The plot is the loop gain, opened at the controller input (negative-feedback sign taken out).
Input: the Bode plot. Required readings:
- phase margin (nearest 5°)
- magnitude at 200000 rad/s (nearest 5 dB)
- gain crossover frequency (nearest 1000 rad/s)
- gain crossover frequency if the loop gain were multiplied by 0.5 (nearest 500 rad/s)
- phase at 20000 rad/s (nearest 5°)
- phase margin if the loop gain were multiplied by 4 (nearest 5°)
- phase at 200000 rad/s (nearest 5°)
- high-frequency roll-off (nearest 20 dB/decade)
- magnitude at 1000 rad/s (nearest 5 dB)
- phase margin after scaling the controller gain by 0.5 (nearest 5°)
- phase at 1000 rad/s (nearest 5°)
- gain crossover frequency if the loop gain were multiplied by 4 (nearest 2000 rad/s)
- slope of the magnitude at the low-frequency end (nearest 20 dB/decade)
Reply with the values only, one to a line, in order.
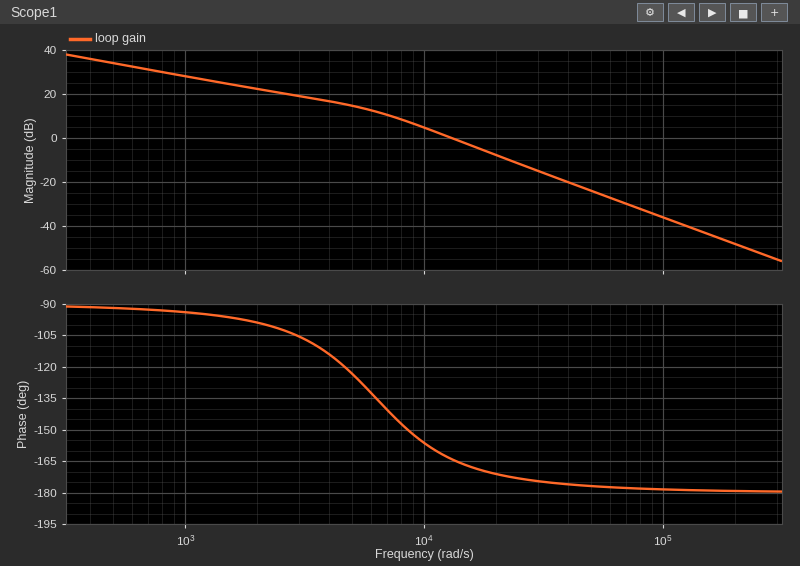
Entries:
15°
-50 dB
13000 rad/s
9500 rad/s
-170°
5°
-180°
-40 dB/decade
30 dB
25°
-95°
26000 rad/s
-20 dB/decade
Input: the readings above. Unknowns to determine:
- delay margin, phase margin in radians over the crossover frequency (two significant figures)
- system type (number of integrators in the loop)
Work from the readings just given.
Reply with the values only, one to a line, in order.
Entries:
0.000020 s
1
